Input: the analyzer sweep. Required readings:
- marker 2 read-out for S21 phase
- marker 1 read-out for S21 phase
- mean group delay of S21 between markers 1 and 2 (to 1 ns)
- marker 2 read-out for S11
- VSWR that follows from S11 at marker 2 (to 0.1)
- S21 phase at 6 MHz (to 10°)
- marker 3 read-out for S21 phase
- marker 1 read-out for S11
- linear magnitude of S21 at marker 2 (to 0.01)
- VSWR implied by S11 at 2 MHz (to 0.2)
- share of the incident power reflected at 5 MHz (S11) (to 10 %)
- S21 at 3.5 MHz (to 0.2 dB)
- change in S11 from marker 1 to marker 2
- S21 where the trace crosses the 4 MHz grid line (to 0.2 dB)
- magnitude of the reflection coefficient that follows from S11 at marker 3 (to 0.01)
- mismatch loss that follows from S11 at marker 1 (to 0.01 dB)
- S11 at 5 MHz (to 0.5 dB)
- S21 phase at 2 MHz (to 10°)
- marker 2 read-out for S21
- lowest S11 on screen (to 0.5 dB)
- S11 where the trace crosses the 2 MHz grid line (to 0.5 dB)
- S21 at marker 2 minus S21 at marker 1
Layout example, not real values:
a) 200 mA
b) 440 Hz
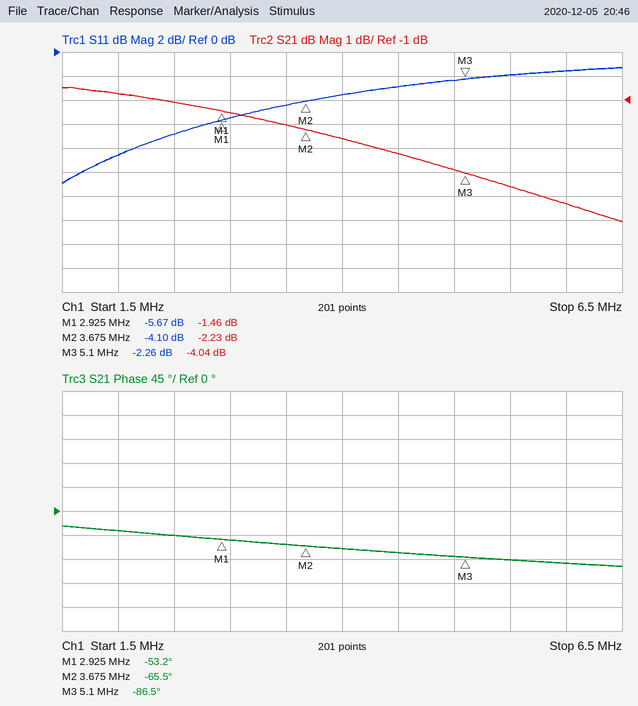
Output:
a) -65.5°
b) -53.2°
c) 46 ns
d) -4.10 dB
e) 4.3
f) -100°
g) -86.5°
h) -5.67 dB
i) 0.77
j) 2.2
k) 60 %
l) -2.0 dB
m) 1.57 dB
n) -2.6 dB
o) 0.77
p) 1.37 dB
q) -2.5 dB
r) -40°
s) -2.23 dB
t) -11.0 dB
u) -8.5 dB
v) -0.77 dB
